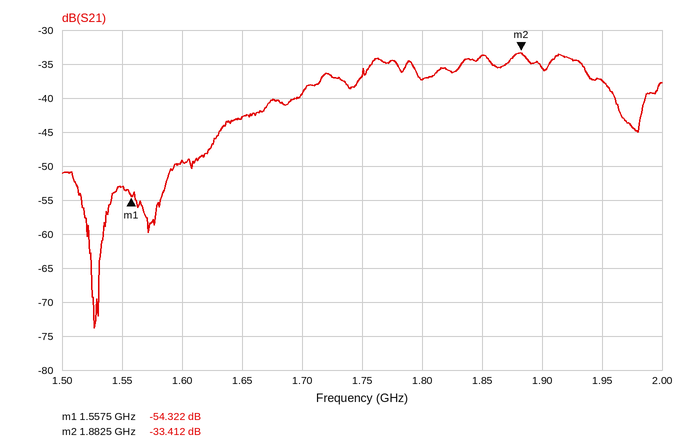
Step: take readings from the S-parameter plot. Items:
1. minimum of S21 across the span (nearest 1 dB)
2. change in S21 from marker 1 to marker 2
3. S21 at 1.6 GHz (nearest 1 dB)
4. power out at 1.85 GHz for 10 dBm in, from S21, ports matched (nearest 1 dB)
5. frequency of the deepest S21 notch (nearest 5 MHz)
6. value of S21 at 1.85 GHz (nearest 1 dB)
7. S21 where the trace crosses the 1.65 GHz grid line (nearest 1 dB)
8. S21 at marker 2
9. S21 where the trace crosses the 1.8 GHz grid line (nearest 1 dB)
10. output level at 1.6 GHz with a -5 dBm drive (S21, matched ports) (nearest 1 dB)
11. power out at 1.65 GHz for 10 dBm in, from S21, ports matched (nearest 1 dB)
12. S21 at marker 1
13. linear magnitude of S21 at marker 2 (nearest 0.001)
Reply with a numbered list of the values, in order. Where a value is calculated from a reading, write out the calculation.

1. -74 dB
2. -33.412 − (-54.322) = 20.910 dB
3. -49 dB
4. 10 dBm + (-34 dB) = -24 dBm
5. 1.525 GHz
6. -34 dB
7. -43 dB
8. -33.412 dB
9. -37 dB
10. -5 dBm + (-49 dB) = -54 dBm
11. 10 dBm + (-43 dB) = -33 dBm
12. -54.322 dB
13. 10^(-33.412/20) ≈ 0.021
